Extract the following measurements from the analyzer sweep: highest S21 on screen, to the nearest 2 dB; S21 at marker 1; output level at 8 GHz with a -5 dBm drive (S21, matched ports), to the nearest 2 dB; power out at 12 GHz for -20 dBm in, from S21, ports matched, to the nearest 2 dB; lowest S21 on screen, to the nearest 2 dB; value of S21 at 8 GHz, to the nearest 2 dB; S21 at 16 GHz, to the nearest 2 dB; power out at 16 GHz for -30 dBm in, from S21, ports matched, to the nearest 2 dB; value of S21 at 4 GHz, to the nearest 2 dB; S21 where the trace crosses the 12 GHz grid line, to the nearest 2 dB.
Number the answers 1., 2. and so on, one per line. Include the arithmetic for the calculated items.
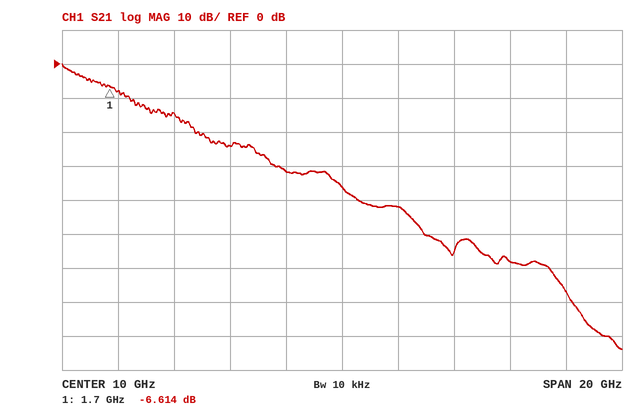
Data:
1. 0 dB
2. -6.614 dB
3. -5 dBm + (-32 dB) = -36 dBm
4. -20 dBm + (-42 dB) = -62 dBm
5. -84 dB
6. -32 dB
7. -58 dB
8. -30 dBm + (-58 dB) = -88 dBm
9. -14 dB
10. -42 dB
